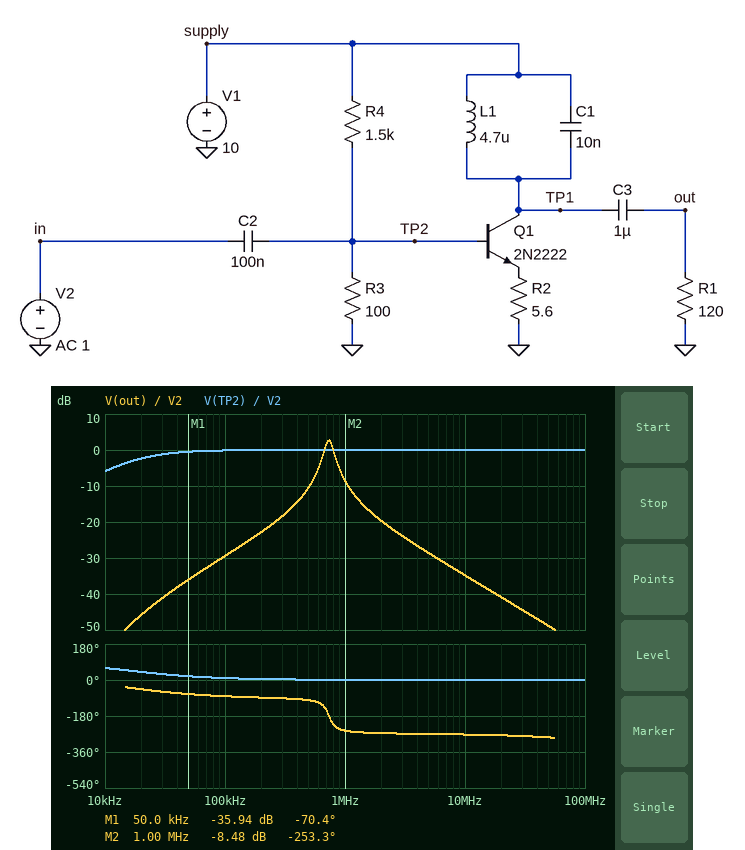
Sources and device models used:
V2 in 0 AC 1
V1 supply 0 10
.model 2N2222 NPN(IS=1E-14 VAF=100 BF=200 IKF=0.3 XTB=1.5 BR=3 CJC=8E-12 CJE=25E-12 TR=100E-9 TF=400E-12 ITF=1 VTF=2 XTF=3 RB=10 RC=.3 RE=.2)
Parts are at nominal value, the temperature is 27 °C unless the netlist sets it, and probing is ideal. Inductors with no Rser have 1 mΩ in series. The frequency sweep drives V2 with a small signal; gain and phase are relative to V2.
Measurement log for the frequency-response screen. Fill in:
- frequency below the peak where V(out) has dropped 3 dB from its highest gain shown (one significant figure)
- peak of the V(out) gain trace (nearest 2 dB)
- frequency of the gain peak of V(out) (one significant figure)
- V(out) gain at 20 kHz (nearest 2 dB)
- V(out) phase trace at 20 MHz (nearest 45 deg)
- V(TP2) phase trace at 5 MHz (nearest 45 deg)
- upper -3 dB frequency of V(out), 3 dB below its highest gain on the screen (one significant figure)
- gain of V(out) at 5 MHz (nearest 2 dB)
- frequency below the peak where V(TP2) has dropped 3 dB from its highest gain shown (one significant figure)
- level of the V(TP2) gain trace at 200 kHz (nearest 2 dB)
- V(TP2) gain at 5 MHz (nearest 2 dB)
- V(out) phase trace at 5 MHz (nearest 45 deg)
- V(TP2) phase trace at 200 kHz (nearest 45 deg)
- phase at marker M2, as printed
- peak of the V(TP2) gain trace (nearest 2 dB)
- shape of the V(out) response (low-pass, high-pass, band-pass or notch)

700 kHz
2 dB
700 kHz
-46 dB
-270 deg
0 deg
800 kHz
-28 dB
20 kHz
0 dB
0 dB
-270 deg
0 deg
-253.3 deg
0 dB
band-pass
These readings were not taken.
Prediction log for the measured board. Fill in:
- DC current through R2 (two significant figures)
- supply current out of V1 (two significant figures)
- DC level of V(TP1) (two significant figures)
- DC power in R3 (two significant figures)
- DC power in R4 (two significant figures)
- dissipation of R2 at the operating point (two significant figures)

320 µA
6.6 mA
10 V
3.9 mW
59 mW
560 nW
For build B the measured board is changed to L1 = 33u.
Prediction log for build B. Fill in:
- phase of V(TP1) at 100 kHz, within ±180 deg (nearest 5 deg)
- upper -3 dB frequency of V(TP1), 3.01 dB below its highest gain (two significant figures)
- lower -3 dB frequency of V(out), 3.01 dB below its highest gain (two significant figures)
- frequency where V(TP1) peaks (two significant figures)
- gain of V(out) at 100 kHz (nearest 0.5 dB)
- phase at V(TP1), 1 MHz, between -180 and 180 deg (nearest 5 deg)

-90 deg
350 kHz
220 kHz
280 kHz
-11.5 dB
100 deg
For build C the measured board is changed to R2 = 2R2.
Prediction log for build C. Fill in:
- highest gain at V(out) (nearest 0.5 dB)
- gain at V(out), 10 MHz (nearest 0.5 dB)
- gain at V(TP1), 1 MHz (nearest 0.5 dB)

3.5 dB
-34.0 dB
-8.0 dB
